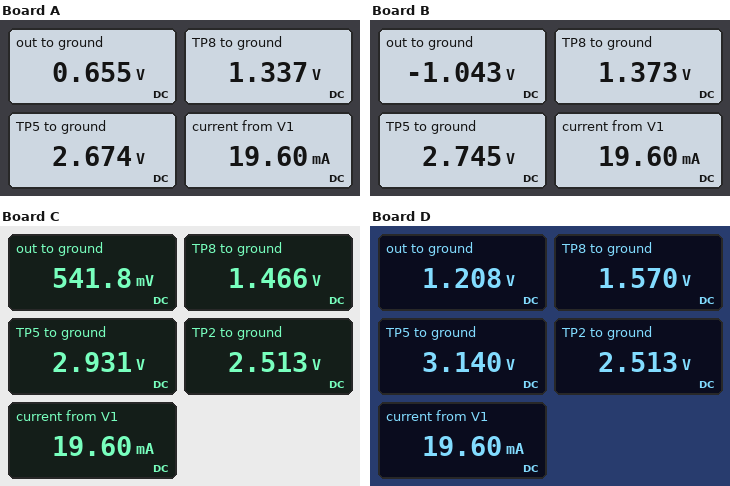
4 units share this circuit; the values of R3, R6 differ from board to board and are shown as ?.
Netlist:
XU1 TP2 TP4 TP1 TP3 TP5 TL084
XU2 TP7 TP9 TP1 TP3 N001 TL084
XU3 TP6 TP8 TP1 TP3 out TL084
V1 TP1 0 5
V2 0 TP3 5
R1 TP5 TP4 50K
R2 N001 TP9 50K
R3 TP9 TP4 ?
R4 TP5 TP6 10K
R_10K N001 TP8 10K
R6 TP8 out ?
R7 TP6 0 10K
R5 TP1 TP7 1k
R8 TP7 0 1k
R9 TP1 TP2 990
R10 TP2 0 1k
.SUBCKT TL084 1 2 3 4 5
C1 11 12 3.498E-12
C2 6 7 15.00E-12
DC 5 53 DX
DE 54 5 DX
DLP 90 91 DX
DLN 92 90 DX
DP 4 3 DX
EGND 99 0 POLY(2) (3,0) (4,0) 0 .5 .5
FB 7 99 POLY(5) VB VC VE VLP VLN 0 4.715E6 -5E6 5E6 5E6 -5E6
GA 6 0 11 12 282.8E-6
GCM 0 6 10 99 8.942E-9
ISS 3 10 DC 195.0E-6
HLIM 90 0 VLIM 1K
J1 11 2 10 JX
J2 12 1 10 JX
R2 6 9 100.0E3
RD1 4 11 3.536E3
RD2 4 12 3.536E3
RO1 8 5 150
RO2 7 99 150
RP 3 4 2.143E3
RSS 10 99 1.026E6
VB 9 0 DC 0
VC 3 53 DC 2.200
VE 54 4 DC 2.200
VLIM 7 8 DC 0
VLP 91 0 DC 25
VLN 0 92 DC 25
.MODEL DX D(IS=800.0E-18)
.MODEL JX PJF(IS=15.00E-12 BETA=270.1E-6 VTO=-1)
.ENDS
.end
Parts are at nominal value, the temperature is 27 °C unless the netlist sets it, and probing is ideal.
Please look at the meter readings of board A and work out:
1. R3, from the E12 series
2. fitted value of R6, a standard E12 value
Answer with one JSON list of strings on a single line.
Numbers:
["3.9 kΩ", "6.8 kΩ"]
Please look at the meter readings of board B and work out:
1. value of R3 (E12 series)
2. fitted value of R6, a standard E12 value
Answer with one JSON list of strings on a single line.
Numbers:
["2.7 kΩ", "27 kΩ"]
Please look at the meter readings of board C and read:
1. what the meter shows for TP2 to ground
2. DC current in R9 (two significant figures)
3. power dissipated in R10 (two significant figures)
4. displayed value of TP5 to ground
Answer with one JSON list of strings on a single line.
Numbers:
["2.513 V", "2.5 mA", "6.3 mW", "2.931 V"]
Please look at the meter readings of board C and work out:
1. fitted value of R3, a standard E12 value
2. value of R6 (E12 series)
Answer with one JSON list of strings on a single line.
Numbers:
["1.5 kΩ", "15 kΩ"]
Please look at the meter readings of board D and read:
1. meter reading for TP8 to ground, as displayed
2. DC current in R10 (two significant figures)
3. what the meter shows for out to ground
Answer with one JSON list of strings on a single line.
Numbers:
["1.570 V", "2.5 mA", "1.208 V"]
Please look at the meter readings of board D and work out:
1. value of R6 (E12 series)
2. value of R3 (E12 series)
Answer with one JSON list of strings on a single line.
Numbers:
["12 kΩ", "1 kΩ"]
